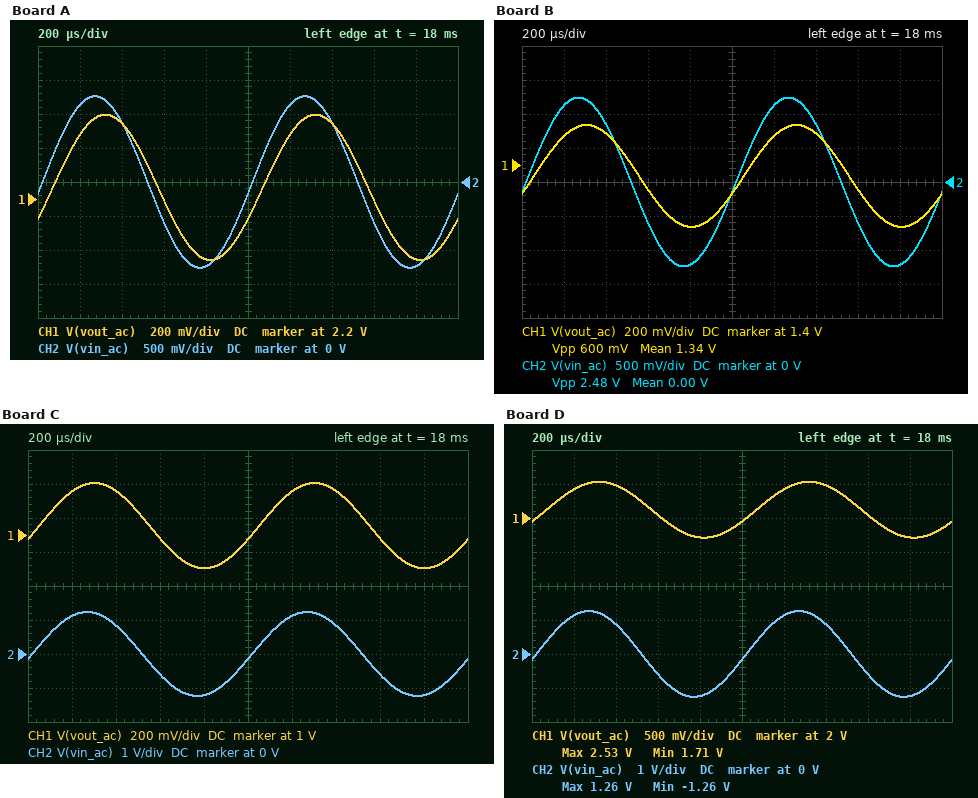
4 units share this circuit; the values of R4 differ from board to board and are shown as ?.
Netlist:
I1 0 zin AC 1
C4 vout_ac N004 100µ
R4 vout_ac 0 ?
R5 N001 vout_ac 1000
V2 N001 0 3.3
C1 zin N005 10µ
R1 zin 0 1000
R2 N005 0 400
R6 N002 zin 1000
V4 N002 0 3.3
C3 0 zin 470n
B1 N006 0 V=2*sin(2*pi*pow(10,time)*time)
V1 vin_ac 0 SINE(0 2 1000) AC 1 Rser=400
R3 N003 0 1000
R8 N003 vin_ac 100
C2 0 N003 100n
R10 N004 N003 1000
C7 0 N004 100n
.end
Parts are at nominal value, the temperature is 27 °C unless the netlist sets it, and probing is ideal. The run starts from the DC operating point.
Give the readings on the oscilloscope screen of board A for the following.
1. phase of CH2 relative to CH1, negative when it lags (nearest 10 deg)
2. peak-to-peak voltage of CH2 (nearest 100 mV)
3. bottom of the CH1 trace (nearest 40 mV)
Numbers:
20 deg
2.5 V
1.84 V
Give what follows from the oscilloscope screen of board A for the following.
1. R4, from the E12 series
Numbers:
2.2 kΩ
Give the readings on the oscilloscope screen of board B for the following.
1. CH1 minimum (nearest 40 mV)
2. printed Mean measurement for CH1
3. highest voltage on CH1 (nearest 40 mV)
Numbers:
1.04 V
1.34 V
1.64 V
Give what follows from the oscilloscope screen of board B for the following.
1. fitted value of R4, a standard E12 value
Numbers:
680 Ω
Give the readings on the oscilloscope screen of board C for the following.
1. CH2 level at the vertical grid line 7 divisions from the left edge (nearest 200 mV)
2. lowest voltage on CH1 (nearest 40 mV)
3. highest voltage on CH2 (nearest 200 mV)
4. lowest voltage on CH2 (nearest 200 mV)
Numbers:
800 mV
800 mV
1.2 V
-1.2 V
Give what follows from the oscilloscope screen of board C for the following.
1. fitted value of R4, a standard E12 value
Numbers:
470 Ω
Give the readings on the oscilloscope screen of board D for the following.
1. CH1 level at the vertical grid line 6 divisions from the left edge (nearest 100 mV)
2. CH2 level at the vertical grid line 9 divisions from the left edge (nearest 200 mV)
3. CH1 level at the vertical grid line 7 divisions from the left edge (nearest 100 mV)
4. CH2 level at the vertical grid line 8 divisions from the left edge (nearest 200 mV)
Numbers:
2.4 V
-1.2 V
2.5 V
-600 mV
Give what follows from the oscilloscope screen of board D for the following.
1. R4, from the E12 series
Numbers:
1.8 kΩ
